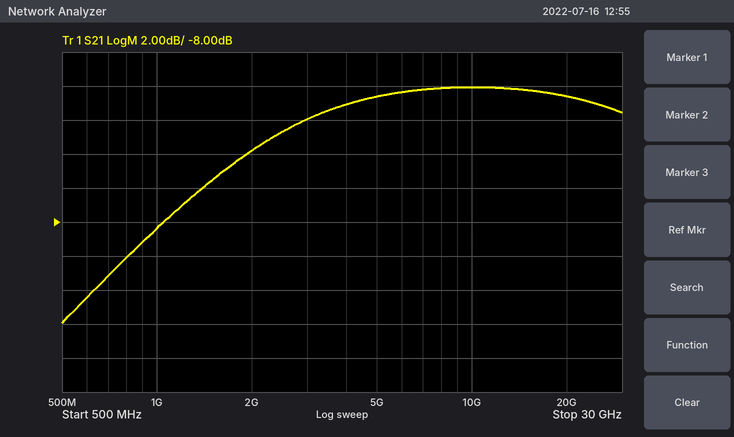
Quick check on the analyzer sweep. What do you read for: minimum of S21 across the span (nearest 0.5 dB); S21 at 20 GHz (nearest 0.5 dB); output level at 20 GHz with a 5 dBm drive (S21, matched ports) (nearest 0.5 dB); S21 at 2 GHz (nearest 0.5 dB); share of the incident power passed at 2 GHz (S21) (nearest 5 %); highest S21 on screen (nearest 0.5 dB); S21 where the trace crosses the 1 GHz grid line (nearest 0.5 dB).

-14.0 dB
-0.5 dB
4.5 dBm
-4.0 dB
40 %
0.0 dB
-8.5 dB
